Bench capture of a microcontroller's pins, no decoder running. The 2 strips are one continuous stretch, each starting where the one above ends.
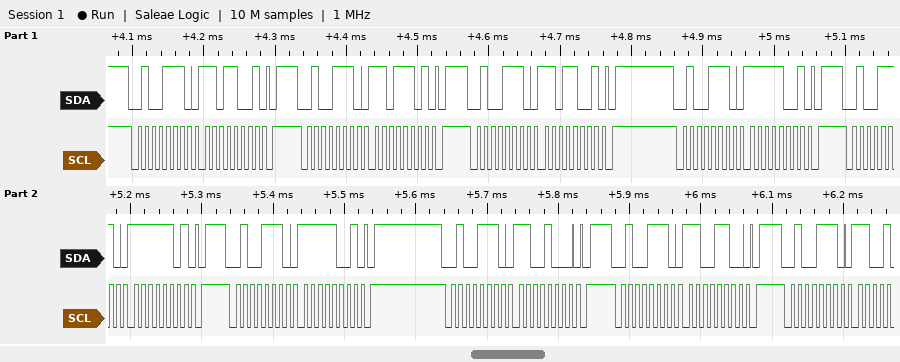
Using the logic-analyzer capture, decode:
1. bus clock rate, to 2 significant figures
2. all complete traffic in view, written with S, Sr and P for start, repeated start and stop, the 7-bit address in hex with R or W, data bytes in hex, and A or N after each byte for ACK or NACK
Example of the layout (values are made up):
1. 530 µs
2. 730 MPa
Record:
1. 100 kHz
2. S 27W A D9 A P S 27W A DD A P S 27W A D9 A P S 27W A F9 A P S 27W A FD A P S 27W A F9 A P S 27W A C8 A P S 27W A CC A P S 27W A
